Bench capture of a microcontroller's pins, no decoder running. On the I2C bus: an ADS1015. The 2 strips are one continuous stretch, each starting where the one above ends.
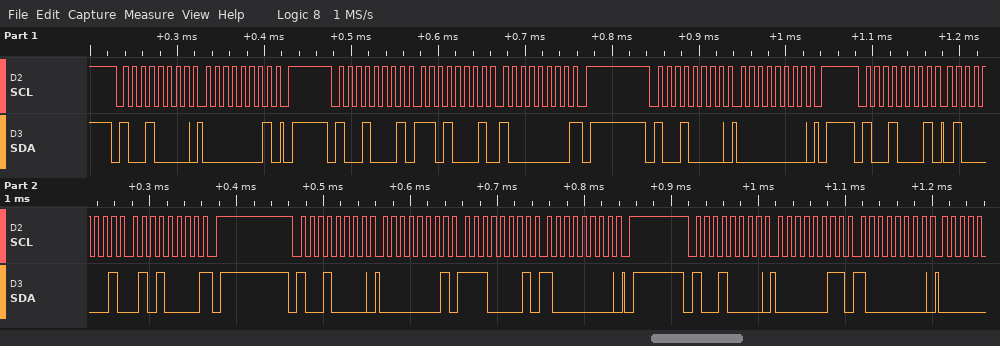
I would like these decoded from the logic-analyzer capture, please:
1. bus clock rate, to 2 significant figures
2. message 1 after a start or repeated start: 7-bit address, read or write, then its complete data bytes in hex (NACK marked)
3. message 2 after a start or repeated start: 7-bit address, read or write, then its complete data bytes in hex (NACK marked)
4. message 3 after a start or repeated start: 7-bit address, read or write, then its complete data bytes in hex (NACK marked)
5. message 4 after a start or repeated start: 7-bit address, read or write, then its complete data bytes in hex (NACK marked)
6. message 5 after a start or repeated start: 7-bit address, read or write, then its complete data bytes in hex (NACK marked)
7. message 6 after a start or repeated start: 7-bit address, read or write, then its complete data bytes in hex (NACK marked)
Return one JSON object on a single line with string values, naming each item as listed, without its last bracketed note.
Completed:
{"bus clock rate, to 2 significant figures": "100 kHz", "message 1 after a start or repeated start: 7-bit address, read or write, then its complete data bytes in hex": "0x48 write: 01", "message 2 after a start or repeated start: 7-bit address, read or write, then its complete data bytes in hex": "0x48 read: D1 80 NACK", "message 3 after a start or repeated start: 7-bit address, read or write, then its complete data bytes in hex": "0x48 write: 00", "message 4 after a start or repeated start: 7-bit address, read or write, then its complete data bytes in hex": "0x48 read: 41 50 NACK", "message 5 after a start or repeated start: 7-bit address, read or write, then its complete data bytes in hex": "0x48 write: 01 E1 80", "message 6 after a start or repeated start: 7-bit address, read or write, then its complete data bytes in hex": "0x48 write: 03 80"}
